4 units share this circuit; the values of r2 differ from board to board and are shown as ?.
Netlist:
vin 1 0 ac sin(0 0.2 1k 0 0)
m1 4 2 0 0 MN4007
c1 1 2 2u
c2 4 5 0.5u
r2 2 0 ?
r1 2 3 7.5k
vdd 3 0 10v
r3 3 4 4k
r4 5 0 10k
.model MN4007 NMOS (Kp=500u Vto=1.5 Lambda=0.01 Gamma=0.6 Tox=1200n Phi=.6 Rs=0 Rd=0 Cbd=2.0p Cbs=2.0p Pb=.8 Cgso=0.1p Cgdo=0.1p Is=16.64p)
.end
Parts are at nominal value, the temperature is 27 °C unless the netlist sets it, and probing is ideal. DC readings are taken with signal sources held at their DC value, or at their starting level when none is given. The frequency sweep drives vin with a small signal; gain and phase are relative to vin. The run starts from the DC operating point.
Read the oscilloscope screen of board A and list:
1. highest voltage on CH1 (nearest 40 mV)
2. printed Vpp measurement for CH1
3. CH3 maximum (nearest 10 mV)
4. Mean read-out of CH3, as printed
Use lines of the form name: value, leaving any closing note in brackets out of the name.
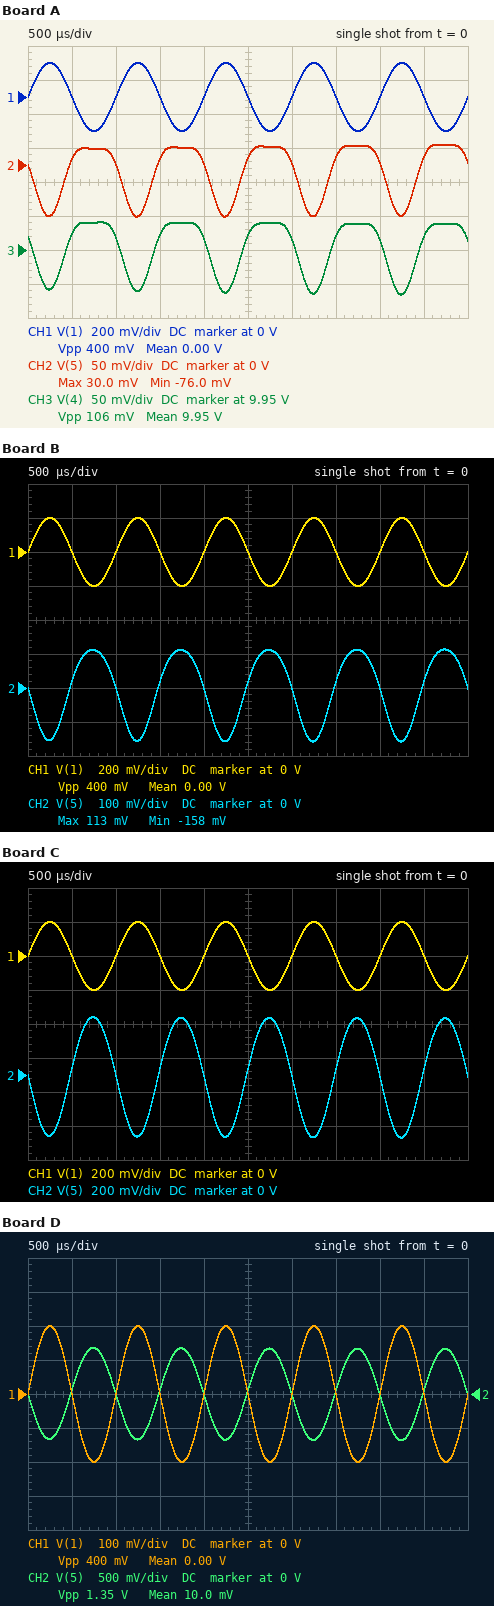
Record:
highest voltage on CH1: 200 mV
printed Vpp measurement for CH1: 400 mV
CH3 maximum: 9.99 V
Mean read-out of CH3, as printed: 9.95 V
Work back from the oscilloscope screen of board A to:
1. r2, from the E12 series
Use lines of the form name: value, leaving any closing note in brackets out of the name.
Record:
r2, from the E12 series: 1.5 kΩ
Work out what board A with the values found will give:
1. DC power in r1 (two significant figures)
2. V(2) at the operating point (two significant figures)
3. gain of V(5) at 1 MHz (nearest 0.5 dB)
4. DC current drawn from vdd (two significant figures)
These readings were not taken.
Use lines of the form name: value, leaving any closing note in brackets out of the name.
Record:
DC power in r1: 9.3 mW
V(2) at the operating point: 1.7 V
gain of V(5) at 1 MHz: -11.5 dB
DC current drawn from vdd: 1.1 mA
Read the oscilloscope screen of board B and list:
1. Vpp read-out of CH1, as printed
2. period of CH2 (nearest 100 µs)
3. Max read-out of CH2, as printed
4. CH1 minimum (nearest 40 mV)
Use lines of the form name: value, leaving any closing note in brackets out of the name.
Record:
Vpp read-out of CH1, as printed: 400 mV
period of CH2: 1.0 ms
Max read-out of CH2, as printed: 113 mV
CH1 minimum: -200 mV
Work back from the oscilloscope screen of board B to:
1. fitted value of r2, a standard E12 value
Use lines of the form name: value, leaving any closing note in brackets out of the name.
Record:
fitted value of r2, a standard E12 value: 1.8 kΩ
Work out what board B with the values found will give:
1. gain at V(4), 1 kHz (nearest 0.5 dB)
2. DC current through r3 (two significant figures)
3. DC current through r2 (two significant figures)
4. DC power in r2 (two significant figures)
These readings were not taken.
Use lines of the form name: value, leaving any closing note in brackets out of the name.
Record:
gain at V(4), 1 kHz: -3.5 dB
DC current through r3: 52 µA
DC current through r2: 1.1 mA
DC power in r2: 2.1 mW
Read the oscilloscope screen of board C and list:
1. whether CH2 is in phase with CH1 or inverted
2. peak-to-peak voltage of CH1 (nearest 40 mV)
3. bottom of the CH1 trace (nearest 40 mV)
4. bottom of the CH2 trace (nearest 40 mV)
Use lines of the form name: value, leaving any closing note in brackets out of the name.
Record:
whether CH2 is in phase with CH1 or inverted: inverted
peak-to-peak voltage of CH1: 400 mV
bottom of the CH1 trace: -200 mV
bottom of the CH2 trace: -360 mV
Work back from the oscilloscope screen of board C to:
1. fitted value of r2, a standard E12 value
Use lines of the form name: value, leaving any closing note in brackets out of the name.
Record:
fitted value of r2, a standard E12 value: 2.7 kΩ
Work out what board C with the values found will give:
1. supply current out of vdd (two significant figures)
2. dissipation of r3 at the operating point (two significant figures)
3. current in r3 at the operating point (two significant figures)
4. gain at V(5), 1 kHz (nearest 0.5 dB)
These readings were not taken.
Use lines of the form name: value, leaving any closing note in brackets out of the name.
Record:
supply current out of vdd: 1.3 mA
dissipation of r3 at the operating point: 510 µW
current in r3 at the operating point: 360 µA
gain at V(5), 1 kHz: 5.0 dB
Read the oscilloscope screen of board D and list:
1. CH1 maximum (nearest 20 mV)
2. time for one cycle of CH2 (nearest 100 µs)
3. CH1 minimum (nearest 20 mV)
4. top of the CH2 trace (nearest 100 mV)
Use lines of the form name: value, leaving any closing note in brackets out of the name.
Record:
CH1 maximum: 200 mV
time for one cycle of CH2: 1.0 ms
CH1 minimum: -200 mV
top of the CH2 trace: 700 mV
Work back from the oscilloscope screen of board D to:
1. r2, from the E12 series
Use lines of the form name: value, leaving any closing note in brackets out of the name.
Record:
r2, from the E12 series: 4.7 kΩ
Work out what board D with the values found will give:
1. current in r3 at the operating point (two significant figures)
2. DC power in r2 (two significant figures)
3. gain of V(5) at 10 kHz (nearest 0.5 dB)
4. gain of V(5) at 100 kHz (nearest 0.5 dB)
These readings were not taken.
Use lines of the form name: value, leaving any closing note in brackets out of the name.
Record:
current in r3 at the operating point: 1.4 mA
DC power in r2: 3.2 mW
gain of V(5) at 10 kHz: 10.5 dB
gain of V(5) at 100 kHz: 10.5 dB
